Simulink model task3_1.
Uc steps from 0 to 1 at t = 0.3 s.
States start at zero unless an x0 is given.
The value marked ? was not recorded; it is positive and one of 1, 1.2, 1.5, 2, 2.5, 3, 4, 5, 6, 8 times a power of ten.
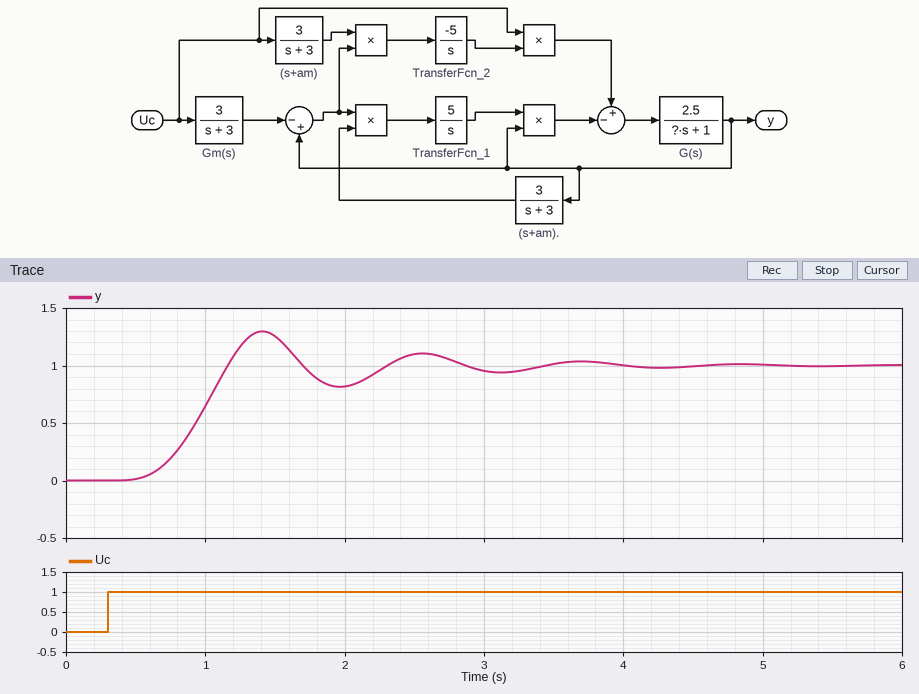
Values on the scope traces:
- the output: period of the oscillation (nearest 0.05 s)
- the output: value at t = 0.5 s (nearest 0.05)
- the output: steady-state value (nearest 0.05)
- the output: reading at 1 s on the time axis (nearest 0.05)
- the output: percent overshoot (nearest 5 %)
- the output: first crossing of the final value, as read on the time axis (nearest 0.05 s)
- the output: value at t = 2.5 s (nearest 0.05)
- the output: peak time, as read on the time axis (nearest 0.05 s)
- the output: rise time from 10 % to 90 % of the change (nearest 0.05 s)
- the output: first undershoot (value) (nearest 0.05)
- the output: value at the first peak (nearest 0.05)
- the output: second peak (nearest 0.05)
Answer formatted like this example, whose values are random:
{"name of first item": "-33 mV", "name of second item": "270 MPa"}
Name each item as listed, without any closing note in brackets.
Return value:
{"the output: period of the oscillation": "1.15 s", "the output: value at t = 0.5 s": "0.00", "the output: steady-state value": "1.00", "the output: reading at 1 s on the time axis": "0.65", "the output: percent overshoot": "30 %", "the output: first crossing of the final value, as read on the time axis": "1.15 s", "the output: value at t = 2.5 s": "1.10", "the output: peak time, as read on the time axis": "1.40 s", "the output: rise time from 10 % to 90 % of the change": "0.45 s", "the output: first undershoot (value)": "0.80", "the output: value at the first peak": "1.30", "the output: second peak": "1.10"}
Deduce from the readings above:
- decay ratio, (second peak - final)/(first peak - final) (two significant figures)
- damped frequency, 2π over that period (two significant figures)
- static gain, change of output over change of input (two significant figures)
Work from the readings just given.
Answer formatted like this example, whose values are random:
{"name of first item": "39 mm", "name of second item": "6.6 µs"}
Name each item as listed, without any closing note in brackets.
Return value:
{"decay ratio, (second peak - final)/(first peak - final)": "0.33", "damped frequency, 2π over that period": "5.5 rad/s", "static gain, change of output over change of input": "1.0"}
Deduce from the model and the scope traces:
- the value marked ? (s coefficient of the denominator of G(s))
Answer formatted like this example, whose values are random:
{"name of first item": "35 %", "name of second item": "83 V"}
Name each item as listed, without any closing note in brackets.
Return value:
{"the value marked ? (s coefficient of the denominator of G(s))": "0.8"}
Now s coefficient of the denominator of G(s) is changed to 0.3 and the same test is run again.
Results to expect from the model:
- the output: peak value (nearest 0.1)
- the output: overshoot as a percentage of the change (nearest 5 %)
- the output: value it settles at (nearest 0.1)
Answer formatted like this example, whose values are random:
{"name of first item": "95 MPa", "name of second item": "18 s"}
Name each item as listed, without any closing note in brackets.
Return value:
{"the output: peak value": "1.1", "the output: overshoot as a percentage of the change": "10 %", "the output: value it settles at": "1.0"}
